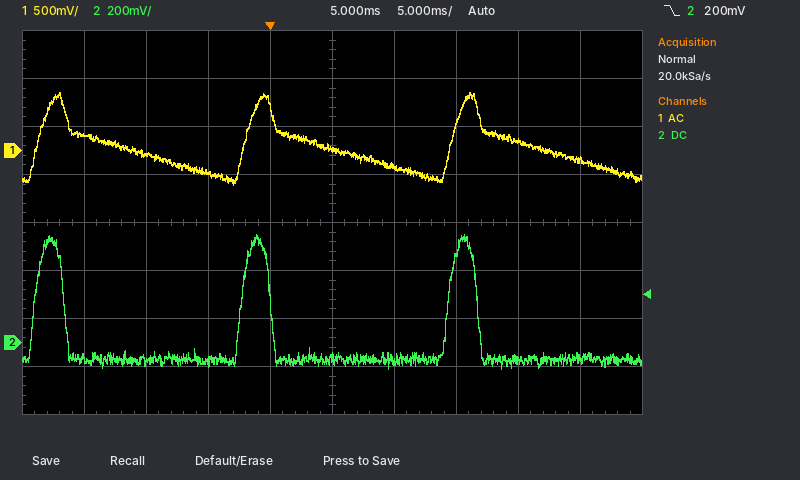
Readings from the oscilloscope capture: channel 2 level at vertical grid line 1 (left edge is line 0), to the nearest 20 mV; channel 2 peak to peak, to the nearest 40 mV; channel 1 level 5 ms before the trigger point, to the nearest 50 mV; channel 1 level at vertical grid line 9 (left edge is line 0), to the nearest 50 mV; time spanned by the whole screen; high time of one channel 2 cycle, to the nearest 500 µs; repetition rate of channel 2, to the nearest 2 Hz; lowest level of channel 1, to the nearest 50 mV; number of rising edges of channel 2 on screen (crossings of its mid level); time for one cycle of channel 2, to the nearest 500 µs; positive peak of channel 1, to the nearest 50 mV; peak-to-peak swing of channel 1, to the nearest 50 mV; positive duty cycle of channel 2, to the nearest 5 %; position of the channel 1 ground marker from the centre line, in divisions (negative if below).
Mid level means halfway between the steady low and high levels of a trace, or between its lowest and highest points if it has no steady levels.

-60 mV
560 mV
-250 mV
-100 mV
50 ms
2.5 ms
60 Hz
-350 mV
3
16.5 ms
600 mV
950 mV
15 %
+1.5 div
